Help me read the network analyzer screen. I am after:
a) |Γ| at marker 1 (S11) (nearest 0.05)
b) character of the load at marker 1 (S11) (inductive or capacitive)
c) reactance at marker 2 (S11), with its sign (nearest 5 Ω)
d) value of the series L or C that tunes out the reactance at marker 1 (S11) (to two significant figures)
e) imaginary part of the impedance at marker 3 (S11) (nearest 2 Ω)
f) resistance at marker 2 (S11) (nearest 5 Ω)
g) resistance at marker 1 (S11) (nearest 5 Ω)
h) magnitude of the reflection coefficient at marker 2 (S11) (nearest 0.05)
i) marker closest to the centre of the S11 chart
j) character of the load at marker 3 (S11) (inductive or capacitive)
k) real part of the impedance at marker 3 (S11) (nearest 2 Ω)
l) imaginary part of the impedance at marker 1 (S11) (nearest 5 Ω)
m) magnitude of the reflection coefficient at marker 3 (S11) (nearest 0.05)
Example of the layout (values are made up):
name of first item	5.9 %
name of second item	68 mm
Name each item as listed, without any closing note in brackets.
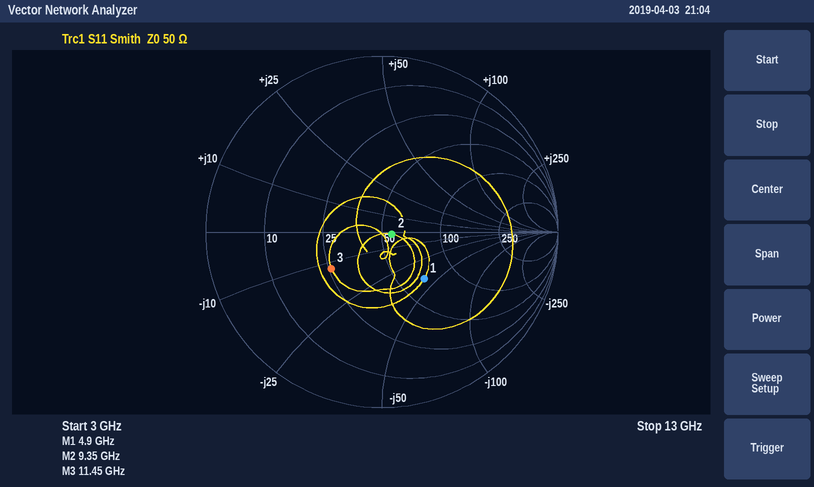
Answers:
|Γ| at marker 1 (S11)	0.35
character of the load at marker 1 (S11)	capacitive
reactance at marker 2 (S11), with its sign	0 Ω
value of the series L or C that tunes out the reactance at marker 1 (S11)	1.3 nH
imaginary part of the impedance at marker 3 (S11)	-12 Ω
resistance at marker 2 (S11)	55 Ω
resistance at marker 1 (S11)	65 Ω
magnitude of the reflection coefficient at marker 2 (S11)	0.05
marker closest to the centre of the S11 chart	marker 2
character of the load at marker 3 (S11)	capacitive
real part of the impedance at marker 3 (S11)	26 Ω
imaginary part of the impedance at marker 1 (S11)	-40 Ω
magnitude of the reflection coefficient at marker 3 (S11)	0.35
